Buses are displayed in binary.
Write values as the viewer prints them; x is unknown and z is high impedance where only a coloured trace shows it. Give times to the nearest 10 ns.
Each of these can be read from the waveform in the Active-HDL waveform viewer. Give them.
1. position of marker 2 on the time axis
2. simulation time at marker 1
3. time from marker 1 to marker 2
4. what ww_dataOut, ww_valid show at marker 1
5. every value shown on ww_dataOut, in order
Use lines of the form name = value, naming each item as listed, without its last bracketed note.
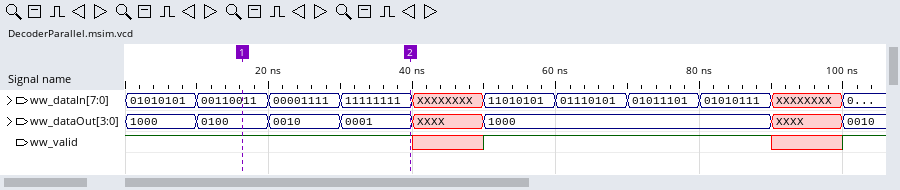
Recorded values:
position of marker 2 on the time axis = 40 ns
simulation time at marker 1 = 20 ns
time from marker 1 to marker 2 = 20 ns
what ww_dataOut, ww_valid show at marker 1 = ww_dataOut=0100, ww_valid=1
every value shown on ww_dataOut, in order = 1000, 0100, 0010, 0001, XXXX, 1000, XXXX, 0010
